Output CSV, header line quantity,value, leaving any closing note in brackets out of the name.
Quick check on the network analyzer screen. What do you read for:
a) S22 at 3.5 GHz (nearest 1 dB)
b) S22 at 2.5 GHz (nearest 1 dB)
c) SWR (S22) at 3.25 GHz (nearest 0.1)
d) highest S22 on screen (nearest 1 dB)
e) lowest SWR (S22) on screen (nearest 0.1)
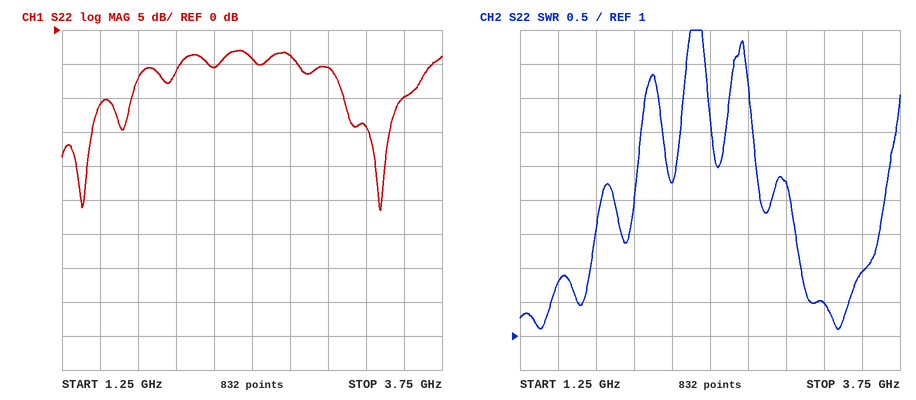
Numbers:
quantity,value
S22 at 3.5 GHz,-10 dB
S22 at 2.5 GHz,-4 dB
SWR (S22) at 3.25 GHz,1.5
highest S22 on screen,-3 dB
lowest SWR (S22) on screen,1.1
